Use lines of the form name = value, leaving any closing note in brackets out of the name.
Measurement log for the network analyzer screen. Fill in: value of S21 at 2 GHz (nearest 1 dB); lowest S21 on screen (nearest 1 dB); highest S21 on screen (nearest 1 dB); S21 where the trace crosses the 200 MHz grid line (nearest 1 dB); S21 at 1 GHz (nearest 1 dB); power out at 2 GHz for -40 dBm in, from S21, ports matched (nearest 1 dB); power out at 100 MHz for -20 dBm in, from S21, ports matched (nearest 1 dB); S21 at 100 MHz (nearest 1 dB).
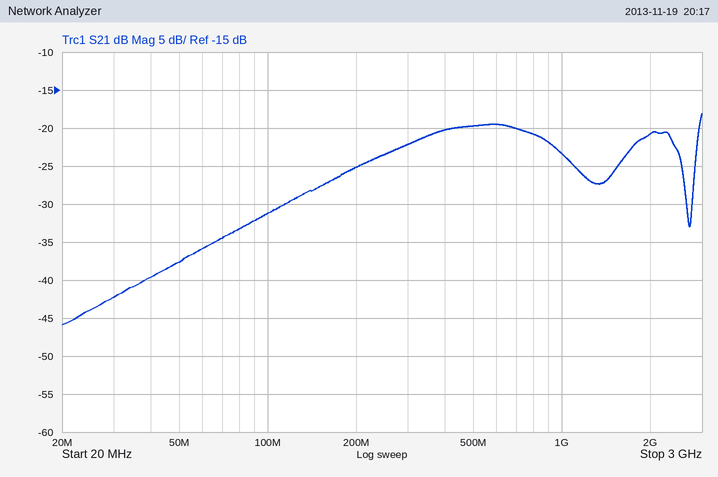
value of S21 at 2 GHz = -21 dB
lowest S21 on screen = -46 dB
highest S21 on screen = -18 dB
S21 where the trace crosses the 200 MHz grid line = -25 dB
S21 at 1 GHz = -23 dB
power out at 2 GHz for -40 dBm in, from S21, ports matched = -61 dBm
power out at 100 MHz for -20 dBm in, from S21, ports matched = -51 dBm
S21 at 100 MHz = -31 dB
